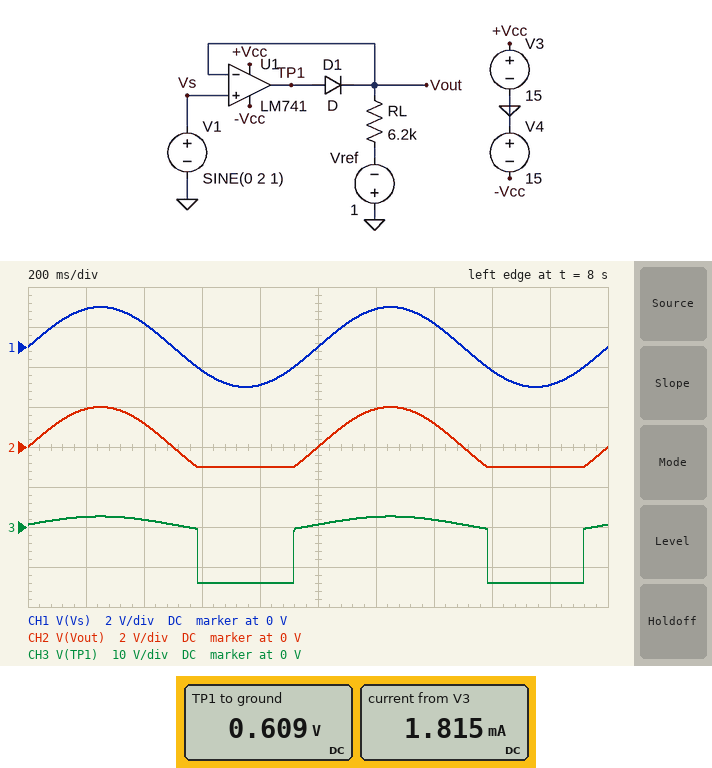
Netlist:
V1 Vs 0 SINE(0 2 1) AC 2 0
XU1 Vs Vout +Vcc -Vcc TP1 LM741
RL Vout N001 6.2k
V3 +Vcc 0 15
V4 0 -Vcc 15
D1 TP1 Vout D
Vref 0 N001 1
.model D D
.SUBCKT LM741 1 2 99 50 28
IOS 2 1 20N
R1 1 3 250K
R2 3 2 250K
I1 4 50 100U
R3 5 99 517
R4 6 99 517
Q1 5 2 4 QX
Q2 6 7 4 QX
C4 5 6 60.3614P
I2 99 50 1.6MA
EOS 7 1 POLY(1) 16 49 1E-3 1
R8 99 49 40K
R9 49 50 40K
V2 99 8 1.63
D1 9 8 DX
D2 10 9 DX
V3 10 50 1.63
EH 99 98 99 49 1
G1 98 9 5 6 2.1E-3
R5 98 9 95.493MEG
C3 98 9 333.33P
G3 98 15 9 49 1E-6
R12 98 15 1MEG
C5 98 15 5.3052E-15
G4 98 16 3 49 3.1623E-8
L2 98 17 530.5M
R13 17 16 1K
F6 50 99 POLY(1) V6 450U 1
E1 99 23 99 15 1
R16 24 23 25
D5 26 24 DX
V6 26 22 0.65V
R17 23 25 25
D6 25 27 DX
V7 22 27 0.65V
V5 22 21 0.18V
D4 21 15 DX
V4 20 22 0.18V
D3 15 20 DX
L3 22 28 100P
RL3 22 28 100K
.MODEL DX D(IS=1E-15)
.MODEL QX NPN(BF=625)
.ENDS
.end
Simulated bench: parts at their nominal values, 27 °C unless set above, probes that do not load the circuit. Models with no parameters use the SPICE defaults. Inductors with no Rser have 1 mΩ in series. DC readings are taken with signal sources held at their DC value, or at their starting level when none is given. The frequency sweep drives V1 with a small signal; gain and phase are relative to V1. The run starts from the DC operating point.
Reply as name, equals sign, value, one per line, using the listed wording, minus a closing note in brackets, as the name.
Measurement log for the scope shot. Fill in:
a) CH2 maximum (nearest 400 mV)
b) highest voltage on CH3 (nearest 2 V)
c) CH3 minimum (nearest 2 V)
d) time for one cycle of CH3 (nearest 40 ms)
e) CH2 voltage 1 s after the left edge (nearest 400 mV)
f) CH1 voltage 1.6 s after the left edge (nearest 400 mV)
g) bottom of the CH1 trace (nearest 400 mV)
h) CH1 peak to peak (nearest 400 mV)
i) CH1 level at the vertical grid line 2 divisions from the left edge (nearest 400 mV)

CH2 maximum = 2.0 V
highest voltage on CH3 = 2 V
CH3 minimum = -14 V
time for one cycle of CH3 = 1.00 s
CH2 voltage 1 s after the left edge = 0 V
CH1 voltage 1.6 s after the left edge = -1.2 V
bottom of the CH1 trace = -2.0 V
CH1 peak to peak = 4.0 V
CH1 level at the vertical grid line 2 divisions from the left edge = 1.2 V
